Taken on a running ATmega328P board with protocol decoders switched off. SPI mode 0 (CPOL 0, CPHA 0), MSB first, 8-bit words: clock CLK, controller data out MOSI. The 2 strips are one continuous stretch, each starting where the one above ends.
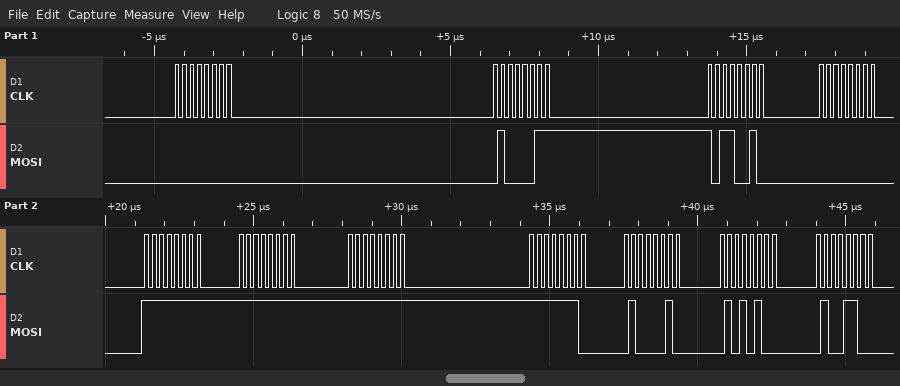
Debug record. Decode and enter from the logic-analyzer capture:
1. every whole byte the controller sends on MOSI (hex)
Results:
00 43 B2 00 FF FF FF FE 42 54 4C
